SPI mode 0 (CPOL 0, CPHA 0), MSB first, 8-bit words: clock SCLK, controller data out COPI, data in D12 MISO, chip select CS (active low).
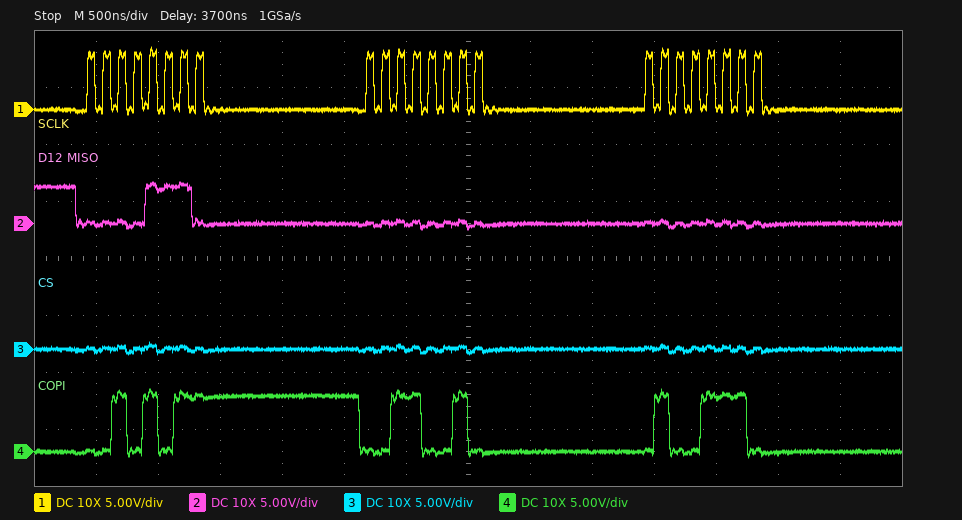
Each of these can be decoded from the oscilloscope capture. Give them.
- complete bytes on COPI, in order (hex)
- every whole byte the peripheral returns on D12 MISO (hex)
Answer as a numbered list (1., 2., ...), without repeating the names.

1. 2B 32 4E
2. 0E 00 00
